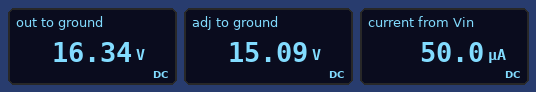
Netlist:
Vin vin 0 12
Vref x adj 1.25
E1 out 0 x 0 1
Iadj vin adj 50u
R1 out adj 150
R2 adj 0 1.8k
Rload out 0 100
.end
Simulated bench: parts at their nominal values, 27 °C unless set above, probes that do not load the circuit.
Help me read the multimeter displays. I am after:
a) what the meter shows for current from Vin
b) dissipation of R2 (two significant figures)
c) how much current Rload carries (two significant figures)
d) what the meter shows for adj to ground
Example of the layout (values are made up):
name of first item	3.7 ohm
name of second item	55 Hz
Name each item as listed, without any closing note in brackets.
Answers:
what the meter shows for current from Vin	50.0 µA
dissipation of R2	130 mW
how much current Rload carries	160 mA
what the meter shows for adj to ground	15.09 V
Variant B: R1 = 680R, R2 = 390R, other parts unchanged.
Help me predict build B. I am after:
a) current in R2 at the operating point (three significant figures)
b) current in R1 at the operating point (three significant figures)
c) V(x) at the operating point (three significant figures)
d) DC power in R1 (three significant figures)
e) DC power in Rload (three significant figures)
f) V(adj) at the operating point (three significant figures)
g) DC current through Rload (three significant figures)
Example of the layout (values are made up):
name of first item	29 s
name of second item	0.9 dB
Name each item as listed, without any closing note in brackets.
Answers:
current in R2 at the operating point	1.89 mA
current in R1 at the operating point	1.84 mA
V(x) at the operating point	1.99 V
DC power in R1	2.30 mW
DC power in Rload	39.5 mW
V(adj) at the operating point	736 mV
DC current through Rload	19.9 mA
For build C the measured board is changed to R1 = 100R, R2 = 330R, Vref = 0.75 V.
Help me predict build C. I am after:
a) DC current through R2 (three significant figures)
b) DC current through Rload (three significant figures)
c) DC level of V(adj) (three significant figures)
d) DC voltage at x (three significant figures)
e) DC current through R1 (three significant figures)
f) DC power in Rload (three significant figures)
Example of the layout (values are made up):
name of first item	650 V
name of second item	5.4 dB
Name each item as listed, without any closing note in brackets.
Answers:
DC current through R2	7.55 mA
DC current through Rload	32.4 mA
DC level of V(adj)	2.49 V
DC voltage at x	3.24 V
DC current through R1	7.50 mA
DC power in Rload	105 mW
